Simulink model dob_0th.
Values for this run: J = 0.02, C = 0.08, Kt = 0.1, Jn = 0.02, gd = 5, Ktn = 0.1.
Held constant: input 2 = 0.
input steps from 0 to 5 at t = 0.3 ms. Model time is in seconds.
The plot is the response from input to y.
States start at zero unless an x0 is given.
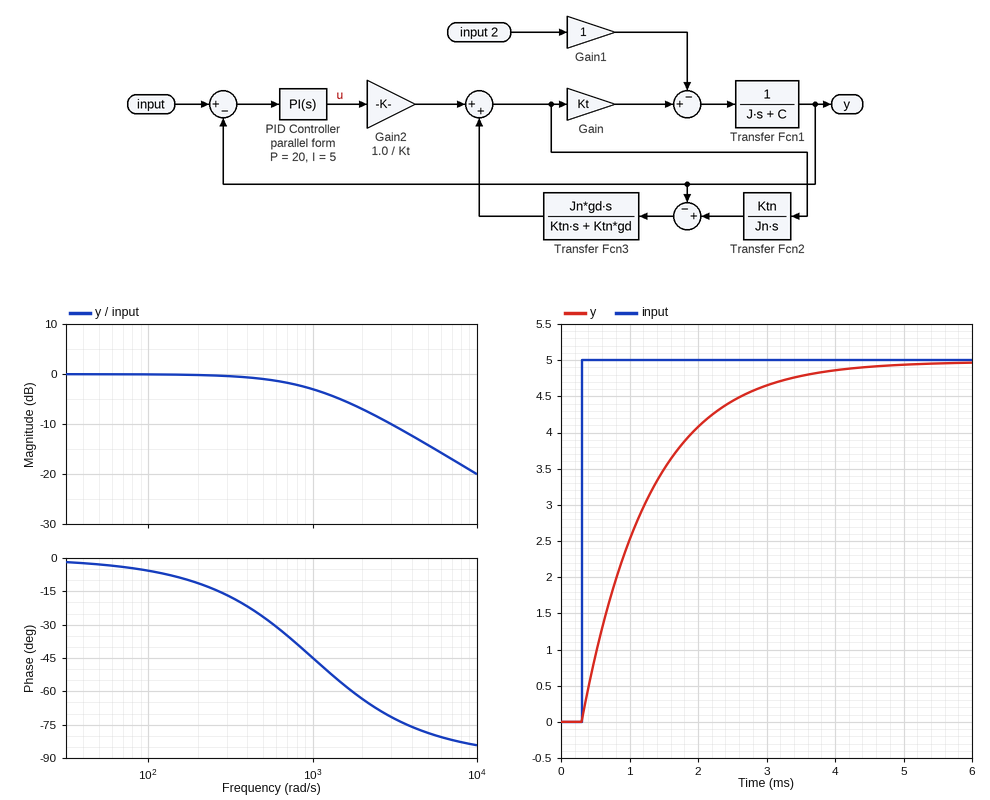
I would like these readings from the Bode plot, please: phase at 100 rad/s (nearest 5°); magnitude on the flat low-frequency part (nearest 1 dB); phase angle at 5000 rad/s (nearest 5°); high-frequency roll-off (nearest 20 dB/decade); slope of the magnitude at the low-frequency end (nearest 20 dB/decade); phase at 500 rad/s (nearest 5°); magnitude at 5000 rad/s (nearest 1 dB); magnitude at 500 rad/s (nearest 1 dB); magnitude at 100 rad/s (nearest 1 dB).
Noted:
-5°
0 dB
-80°
-20 dB/decade
0 dB/decade
-25°
-14 dB
-1 dB
0 dB
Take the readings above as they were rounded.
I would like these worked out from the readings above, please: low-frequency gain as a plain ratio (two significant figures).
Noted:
1.0
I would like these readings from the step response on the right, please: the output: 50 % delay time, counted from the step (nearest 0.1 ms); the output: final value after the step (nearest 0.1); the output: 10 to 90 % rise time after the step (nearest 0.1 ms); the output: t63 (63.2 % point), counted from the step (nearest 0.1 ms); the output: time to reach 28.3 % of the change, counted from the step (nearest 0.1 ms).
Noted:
0.7 ms
5.0
2.2 ms
1.0 ms
0.3 ms
